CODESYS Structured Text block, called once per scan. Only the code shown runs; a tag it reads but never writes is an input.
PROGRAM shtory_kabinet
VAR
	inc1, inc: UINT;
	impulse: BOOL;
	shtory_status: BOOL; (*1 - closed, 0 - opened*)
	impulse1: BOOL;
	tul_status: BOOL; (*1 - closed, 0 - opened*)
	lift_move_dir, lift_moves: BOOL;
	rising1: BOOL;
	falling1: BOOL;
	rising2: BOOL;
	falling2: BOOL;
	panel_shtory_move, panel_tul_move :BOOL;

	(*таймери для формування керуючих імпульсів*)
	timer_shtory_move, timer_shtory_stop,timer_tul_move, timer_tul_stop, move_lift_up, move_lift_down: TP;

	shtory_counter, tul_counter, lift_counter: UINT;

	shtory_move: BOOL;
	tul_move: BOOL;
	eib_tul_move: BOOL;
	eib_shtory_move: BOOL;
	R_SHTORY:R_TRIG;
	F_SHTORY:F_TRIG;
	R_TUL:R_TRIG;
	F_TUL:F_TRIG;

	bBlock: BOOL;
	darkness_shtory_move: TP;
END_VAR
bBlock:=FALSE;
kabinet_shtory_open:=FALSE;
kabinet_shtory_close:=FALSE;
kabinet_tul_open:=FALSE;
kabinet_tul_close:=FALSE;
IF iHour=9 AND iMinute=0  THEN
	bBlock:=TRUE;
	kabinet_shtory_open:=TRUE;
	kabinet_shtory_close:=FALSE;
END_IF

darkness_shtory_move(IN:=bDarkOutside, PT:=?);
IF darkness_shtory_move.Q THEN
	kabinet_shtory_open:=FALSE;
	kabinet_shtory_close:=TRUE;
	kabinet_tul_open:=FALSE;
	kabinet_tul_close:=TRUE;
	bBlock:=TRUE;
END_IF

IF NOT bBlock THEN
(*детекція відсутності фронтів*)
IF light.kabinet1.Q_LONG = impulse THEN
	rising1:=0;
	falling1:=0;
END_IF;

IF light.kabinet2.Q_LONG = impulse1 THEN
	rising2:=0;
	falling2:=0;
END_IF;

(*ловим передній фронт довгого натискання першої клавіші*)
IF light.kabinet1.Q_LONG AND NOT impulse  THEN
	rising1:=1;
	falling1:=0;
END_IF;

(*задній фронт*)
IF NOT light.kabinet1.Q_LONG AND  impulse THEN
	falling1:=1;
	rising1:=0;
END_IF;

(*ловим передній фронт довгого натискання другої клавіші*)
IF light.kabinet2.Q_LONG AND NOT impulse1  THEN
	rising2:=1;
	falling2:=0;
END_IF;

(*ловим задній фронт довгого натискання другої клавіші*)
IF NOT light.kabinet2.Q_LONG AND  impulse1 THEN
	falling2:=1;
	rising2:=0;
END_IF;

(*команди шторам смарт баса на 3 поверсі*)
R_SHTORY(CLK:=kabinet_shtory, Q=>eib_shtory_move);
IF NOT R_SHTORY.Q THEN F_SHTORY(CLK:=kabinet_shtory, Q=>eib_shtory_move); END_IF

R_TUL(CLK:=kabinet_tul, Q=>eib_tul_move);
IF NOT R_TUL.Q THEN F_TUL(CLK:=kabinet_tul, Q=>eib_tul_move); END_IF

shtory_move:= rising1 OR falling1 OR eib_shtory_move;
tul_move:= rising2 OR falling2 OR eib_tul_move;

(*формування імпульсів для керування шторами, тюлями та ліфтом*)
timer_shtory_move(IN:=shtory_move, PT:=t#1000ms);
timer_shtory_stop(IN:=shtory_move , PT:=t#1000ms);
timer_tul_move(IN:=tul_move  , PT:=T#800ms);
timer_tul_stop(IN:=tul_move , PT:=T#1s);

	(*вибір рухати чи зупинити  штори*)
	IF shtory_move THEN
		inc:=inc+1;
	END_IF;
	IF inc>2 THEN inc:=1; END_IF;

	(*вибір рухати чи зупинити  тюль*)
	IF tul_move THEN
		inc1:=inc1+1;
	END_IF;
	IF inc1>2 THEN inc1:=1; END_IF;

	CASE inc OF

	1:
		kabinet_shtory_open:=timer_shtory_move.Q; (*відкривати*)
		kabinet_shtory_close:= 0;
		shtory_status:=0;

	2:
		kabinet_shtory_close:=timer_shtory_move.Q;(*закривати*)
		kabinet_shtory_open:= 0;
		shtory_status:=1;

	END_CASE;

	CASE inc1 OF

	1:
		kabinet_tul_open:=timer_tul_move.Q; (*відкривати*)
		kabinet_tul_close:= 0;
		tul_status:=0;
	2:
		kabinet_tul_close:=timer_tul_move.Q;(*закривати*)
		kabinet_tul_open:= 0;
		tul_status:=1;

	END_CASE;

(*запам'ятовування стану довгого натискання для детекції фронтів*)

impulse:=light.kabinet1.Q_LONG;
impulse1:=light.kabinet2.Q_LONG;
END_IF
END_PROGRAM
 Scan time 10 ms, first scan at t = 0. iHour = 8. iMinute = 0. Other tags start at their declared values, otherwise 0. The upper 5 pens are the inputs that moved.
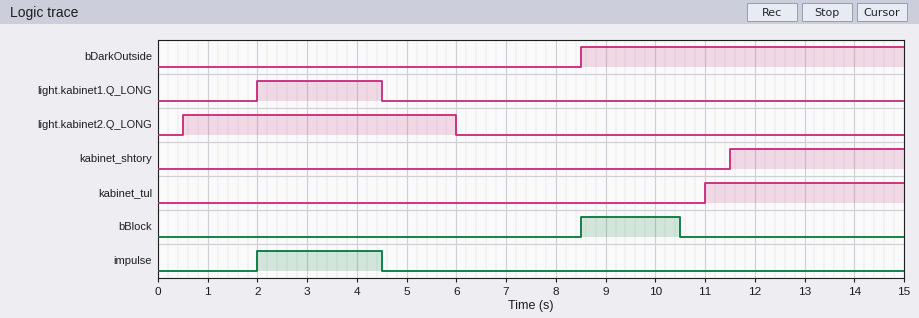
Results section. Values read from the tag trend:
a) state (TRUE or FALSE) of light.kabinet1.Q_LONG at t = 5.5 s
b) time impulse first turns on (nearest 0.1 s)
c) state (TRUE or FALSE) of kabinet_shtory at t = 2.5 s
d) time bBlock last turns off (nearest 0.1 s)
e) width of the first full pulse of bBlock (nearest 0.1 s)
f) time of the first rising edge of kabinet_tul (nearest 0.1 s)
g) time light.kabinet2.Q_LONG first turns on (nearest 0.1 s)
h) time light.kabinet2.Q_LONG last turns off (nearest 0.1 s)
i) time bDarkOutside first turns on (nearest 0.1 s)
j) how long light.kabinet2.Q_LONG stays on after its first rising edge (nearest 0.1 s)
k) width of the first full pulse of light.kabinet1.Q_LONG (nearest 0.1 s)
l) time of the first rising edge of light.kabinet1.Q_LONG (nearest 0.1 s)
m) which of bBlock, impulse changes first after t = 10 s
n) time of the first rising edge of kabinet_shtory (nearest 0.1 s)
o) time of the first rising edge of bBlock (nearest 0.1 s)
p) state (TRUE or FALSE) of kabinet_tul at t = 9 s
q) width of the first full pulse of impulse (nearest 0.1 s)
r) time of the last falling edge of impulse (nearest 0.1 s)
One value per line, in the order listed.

FALSE
2.0 s
FALSE
10.5 s
2.0 s
11.0 s
0.5 s
6.0 s
8.5 s
5.5 s
2.5 s
2.0 s
bBlock
11.5 s
8.5 s
FALSE
2.5 s
4.5 s
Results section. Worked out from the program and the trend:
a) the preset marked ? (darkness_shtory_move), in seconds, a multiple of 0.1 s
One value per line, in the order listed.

2.0 s
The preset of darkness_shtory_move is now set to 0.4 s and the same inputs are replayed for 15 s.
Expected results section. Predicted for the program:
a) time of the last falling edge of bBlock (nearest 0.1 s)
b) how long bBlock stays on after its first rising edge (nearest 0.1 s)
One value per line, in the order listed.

8.9 s
0.4 s
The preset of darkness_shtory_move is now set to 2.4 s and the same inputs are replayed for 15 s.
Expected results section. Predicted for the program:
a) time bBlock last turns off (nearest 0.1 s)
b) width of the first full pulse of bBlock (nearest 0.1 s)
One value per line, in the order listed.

10.9 s
2.4 s
